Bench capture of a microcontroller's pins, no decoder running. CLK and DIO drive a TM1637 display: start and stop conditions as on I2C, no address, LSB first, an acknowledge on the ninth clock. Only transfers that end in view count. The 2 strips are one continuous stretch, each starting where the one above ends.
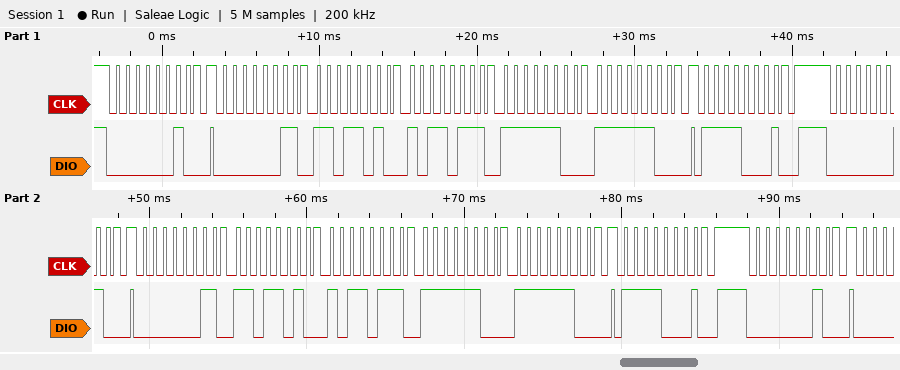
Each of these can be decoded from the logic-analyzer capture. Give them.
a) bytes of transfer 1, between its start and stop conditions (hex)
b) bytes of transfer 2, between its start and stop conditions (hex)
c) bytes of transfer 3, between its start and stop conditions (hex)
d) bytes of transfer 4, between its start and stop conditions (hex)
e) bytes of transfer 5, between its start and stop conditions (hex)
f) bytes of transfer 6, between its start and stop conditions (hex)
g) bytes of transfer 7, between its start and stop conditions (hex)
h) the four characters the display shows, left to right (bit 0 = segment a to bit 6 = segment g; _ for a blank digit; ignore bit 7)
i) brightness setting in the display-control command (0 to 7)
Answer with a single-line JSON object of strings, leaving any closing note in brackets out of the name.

{"bytes of transfer 1, between its start and stop conditions": "40", "bytes of transfer 2, between its start and stop conditions": "C0 5B ED 3F 3F", "bytes of transfer 3, between its start and stop conditions": "8F", "bytes of transfer 4, between its start and stop conditions": "40", "bytes of transfer 5, between its start and stop conditions": "C0 5B ED 3F 3F", "bytes of transfer 6, between its start and stop conditions": "8F", "bytes of transfer 7, between its start and stop conditions": "40", "the four characters the display shows, left to right": "2500", "brightness setting in the display-control command": "7"}
